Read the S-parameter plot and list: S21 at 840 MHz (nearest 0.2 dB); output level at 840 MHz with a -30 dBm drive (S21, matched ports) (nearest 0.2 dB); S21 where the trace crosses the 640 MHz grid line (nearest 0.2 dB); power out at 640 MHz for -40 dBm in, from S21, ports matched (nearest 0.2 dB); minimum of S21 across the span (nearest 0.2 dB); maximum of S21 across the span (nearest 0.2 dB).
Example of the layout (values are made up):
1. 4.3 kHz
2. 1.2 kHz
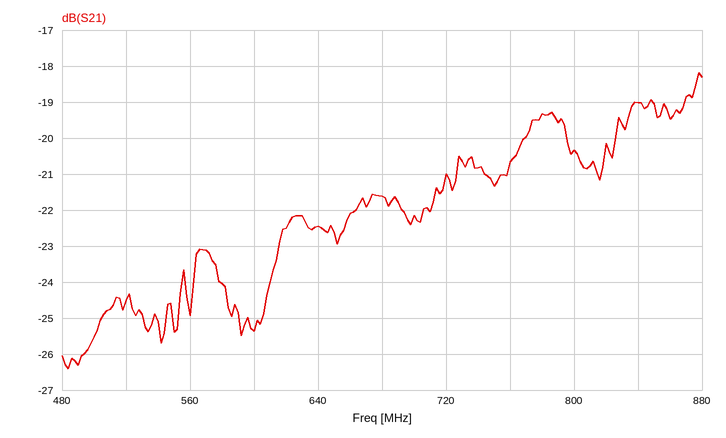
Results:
1. -19.0 dB
2. -49.0 dBm
3. -22.4 dB
4. -62.4 dBm
5. -26.4 dB
6. -18.2 dB
